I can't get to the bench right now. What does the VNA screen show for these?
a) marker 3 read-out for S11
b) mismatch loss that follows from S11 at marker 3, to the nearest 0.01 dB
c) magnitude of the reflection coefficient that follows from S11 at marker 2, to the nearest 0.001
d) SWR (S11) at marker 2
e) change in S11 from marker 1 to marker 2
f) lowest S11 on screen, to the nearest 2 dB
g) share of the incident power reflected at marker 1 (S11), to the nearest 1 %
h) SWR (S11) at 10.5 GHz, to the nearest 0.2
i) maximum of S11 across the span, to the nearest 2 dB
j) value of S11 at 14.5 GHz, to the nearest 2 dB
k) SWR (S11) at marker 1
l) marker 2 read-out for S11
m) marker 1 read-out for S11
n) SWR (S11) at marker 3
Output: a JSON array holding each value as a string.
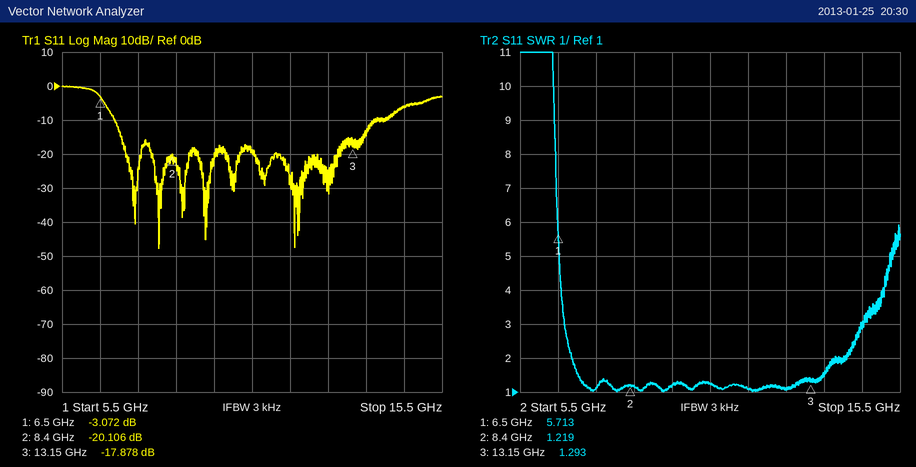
["-17.878 dB", "0.07 dB", "0.099", "1.219", "-17.034 dB", "-48 dB", "49 %", "1.2", "0 dB", "-6 dB", "5.713", "-20.106 dB", "-3.072 dB", "1.293"]
